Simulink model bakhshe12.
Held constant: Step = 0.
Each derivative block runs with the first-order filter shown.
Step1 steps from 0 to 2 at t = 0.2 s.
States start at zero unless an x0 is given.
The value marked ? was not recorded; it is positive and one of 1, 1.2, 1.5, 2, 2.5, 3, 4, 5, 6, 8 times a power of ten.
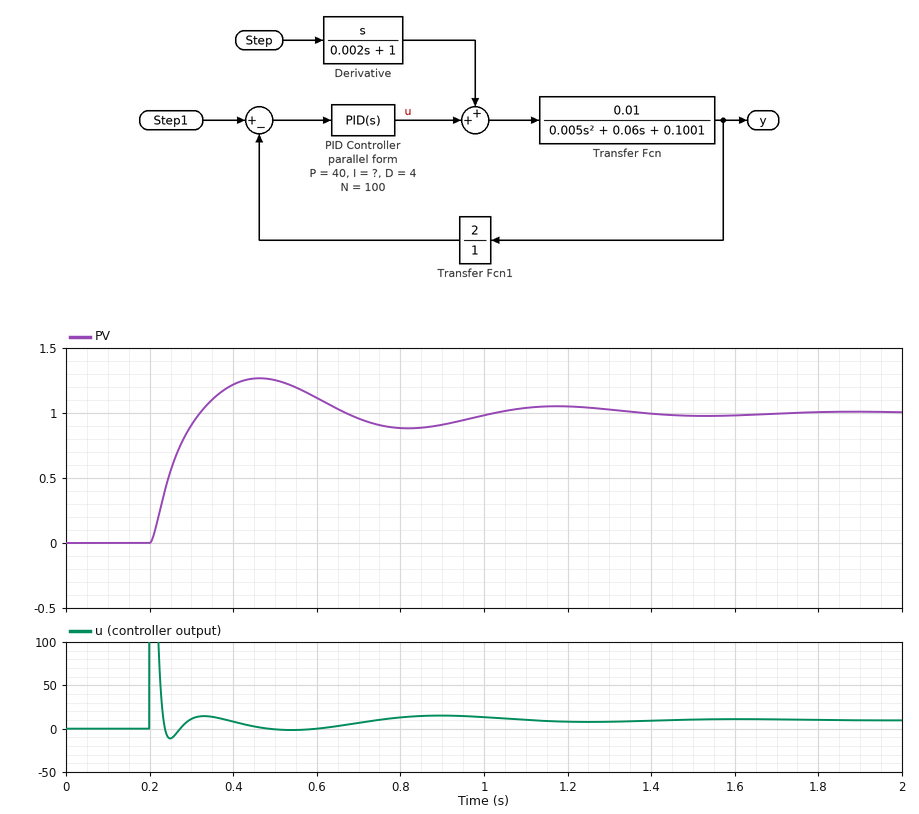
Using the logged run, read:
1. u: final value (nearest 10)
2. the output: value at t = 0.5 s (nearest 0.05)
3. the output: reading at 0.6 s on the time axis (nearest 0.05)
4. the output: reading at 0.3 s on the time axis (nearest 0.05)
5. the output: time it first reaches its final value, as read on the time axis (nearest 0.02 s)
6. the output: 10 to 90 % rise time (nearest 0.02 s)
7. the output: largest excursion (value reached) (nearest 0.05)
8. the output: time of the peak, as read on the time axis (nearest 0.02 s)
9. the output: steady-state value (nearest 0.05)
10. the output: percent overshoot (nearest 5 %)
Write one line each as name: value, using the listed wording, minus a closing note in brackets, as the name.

u: final value: 10
the output: value at t = 0.5 s: 1.25
the output: reading at 0.6 s on the time axis: 1.10
the output: reading at 0.3 s on the time axis: 0.90
the output: time it first reaches its final value, as read on the time axis: 0.32 s
the output: 10 to 90 % rise time: 0.08 s
the output: largest excursion (value reached): 1.25
the output: time of the peak, as read on the time axis: 0.46 s
the output: steady-state value: 1.00
the output: percent overshoot: 25 %
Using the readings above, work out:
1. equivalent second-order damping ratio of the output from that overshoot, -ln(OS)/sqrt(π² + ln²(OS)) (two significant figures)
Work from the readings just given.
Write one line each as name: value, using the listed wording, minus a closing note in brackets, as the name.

equivalent second-order damping ratio of the output from that overshoot, -ln(OS)/sqrt(π² + ln²(OS)): 0.40
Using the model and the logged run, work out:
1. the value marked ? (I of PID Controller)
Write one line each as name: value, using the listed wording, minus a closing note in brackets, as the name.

the value marked ?: 500
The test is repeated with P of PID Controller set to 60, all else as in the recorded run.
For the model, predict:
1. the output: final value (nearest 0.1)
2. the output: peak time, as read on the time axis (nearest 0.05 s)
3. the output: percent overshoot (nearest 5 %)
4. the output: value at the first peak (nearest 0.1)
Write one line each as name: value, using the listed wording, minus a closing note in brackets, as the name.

the output: final value: 1.0
the output: peak time, as read on the time axis: 0.40 s
the output: percent overshoot: 20 %
the output: value at the first peak: 1.2
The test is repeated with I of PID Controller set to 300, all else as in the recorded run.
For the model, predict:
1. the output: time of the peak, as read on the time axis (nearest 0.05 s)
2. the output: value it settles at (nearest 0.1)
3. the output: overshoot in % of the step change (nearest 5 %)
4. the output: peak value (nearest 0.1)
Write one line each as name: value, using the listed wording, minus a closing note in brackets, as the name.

the output: time of the peak, as read on the time axis: 0.50 s
the output: value it settles at: 1.0
the output: overshoot in % of the step change: 15 %
the output: peak value: 1.2
